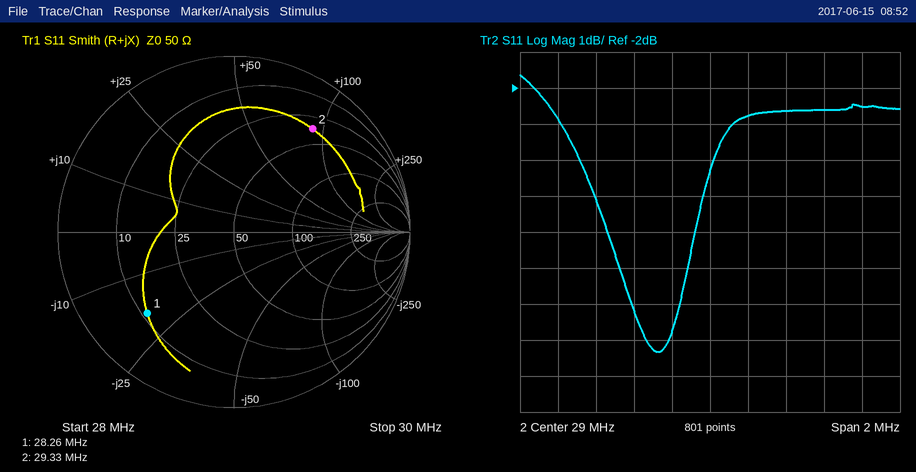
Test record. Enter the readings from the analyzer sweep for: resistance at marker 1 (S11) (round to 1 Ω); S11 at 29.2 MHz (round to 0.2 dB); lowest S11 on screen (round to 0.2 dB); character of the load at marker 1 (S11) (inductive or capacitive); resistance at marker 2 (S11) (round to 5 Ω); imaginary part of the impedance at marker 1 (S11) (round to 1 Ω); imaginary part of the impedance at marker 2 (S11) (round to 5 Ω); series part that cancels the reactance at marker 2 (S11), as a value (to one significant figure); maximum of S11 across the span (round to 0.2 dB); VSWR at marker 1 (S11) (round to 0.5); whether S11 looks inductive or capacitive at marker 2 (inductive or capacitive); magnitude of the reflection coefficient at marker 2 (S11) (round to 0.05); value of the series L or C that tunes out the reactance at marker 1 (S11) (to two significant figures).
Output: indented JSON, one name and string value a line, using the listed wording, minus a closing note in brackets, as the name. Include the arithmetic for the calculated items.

{
  "resistance at marker 1 (S11)": "11 Ω",
  "S11 at 29.2 MHz": "-2.8 dB",
  "lowest S11 on screen": "-9.4 dB",
  "character of the load at marker 1 (S11)": "capacitive",
  "resistance at marker 2 (S11)": "35 Ω",
  "imaginary part of the impedance at marker 1 (S11)": "-19 Ω",
  "imaginary part of the impedance at marker 2 (S11)": "+90 Ω",
  "series part that cancels the reactance at marker 2 (S11), as a value": "C = 1/(2π × 29.33 MHz × 90 Ω) ≈ 60 pF",
  "maximum of S11 across the span": "-1.6 dB",
  "VSWR at marker 1 (S11)": "5.0",
  "whether S11 looks inductive or capacitive at marker 2": "inductive",
  "magnitude of the reflection coefficient at marker 2 (S11)": "0.75",
  "value of the series L or C that tunes out the reactance at marker 1 (S11)": "L = 19 Ω/(2π × 28.26 MHz) ≈ 107 nH, so 110 nH to two significant figures"
}
